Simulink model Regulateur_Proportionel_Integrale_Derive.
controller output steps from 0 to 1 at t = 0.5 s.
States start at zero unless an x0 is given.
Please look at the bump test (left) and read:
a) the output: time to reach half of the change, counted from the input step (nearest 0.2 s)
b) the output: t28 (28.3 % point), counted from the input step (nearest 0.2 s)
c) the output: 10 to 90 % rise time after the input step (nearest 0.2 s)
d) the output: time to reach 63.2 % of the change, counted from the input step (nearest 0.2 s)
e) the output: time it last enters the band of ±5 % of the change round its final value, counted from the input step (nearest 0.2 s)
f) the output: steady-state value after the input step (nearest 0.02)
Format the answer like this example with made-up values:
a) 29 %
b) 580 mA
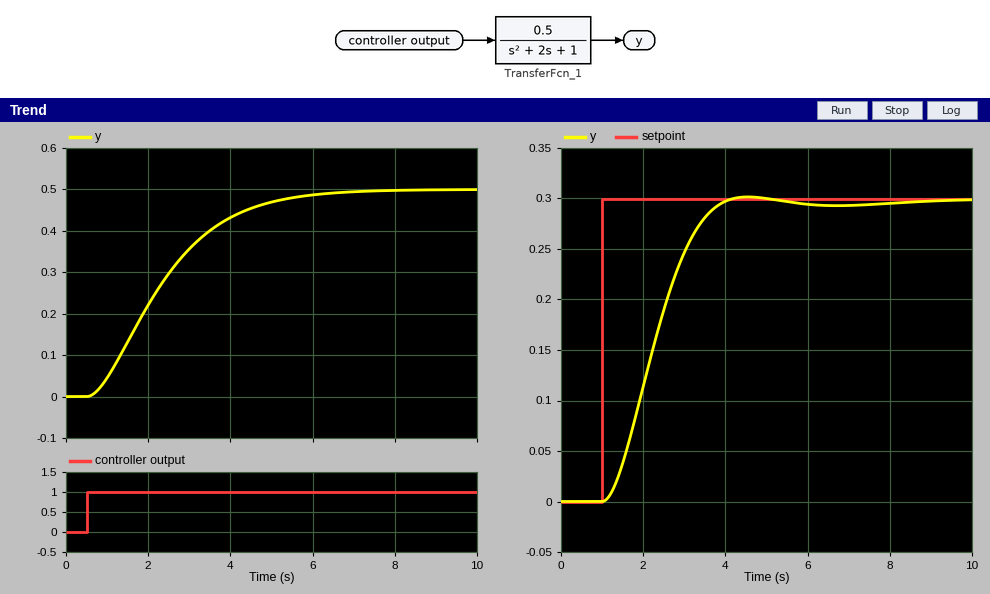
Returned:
a) 1.6 s
b) 1.0 s
c) 3.4 s
d) 2.2 s
e) 4.8 s
f) 0.50
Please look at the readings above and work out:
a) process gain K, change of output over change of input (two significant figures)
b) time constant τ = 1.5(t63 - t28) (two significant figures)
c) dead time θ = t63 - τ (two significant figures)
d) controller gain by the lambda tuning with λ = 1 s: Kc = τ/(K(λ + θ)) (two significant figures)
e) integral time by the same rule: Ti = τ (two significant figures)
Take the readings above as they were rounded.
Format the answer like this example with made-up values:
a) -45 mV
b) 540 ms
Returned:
a) 0.50
b) 1.8 s
c) 0.40 s
d) 2.6
e) 1.8 s
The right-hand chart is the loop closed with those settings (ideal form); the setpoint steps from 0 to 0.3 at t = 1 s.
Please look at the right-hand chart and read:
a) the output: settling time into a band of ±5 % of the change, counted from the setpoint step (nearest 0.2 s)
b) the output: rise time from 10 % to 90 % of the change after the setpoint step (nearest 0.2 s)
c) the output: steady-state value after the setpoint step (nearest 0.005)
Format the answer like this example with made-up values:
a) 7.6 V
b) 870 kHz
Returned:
a) 2.6 s
b) 1.8 s
c) 0.300
